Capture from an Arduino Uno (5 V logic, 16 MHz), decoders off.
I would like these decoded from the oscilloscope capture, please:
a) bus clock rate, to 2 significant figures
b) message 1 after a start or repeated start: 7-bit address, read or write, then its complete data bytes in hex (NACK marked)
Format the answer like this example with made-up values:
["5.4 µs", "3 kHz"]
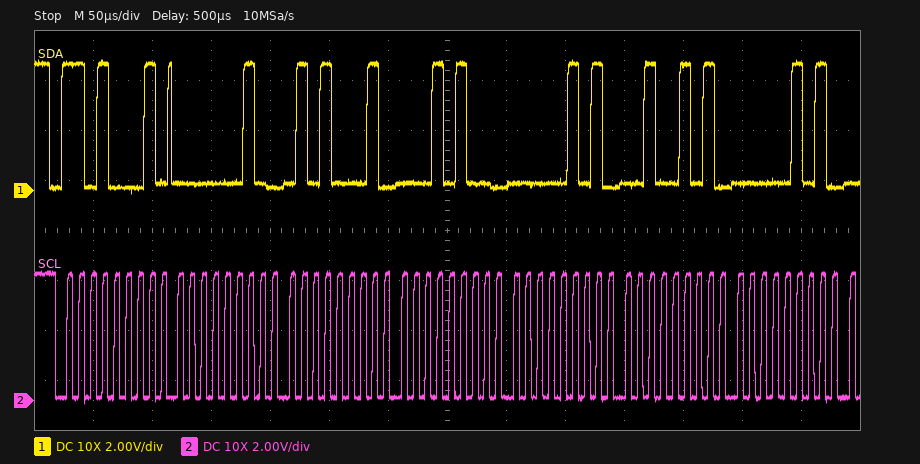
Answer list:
["100 kHz", "0x68 read: 02 51 14 05 25 05"]
